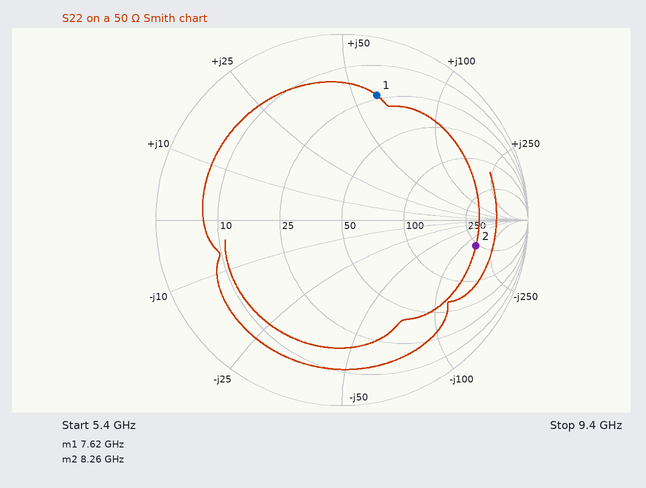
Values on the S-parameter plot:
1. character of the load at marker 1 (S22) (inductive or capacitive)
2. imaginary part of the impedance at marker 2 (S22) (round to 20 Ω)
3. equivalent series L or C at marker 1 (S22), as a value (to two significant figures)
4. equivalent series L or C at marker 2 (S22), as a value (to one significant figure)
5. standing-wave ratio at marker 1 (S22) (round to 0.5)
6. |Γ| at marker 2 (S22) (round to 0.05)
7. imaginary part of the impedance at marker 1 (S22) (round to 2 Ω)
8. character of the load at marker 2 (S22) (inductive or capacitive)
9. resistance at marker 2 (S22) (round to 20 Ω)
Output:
inductive
-140 Ω
1.3 nH
100 fF
5.5
0.75
+60 Ω
capacitive
240 Ω
